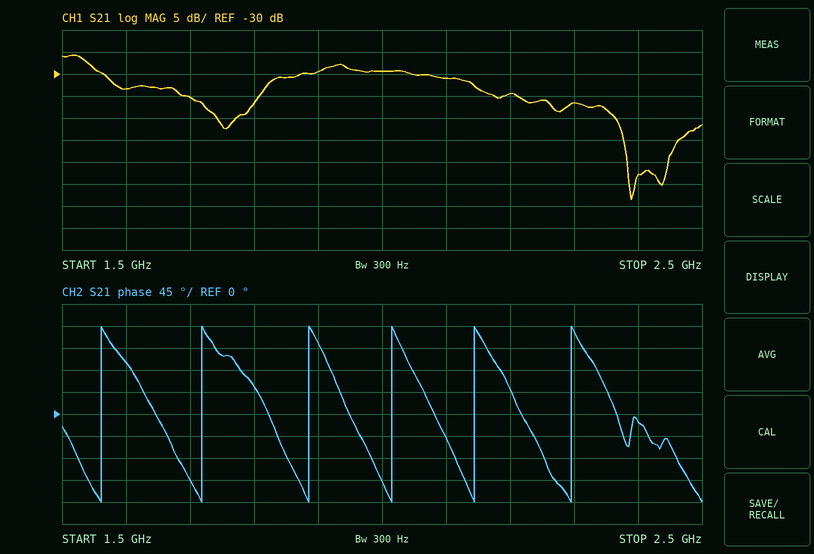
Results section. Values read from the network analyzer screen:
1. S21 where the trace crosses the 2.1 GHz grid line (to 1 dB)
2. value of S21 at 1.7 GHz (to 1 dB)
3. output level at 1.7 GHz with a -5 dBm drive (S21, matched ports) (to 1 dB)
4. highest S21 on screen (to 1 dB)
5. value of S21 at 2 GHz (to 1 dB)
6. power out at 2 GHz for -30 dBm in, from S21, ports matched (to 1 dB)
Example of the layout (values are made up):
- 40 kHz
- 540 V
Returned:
- -31 dB
- -35 dB
- -40 dBm
- -26 dB
- -29 dB
- -59 dBm
